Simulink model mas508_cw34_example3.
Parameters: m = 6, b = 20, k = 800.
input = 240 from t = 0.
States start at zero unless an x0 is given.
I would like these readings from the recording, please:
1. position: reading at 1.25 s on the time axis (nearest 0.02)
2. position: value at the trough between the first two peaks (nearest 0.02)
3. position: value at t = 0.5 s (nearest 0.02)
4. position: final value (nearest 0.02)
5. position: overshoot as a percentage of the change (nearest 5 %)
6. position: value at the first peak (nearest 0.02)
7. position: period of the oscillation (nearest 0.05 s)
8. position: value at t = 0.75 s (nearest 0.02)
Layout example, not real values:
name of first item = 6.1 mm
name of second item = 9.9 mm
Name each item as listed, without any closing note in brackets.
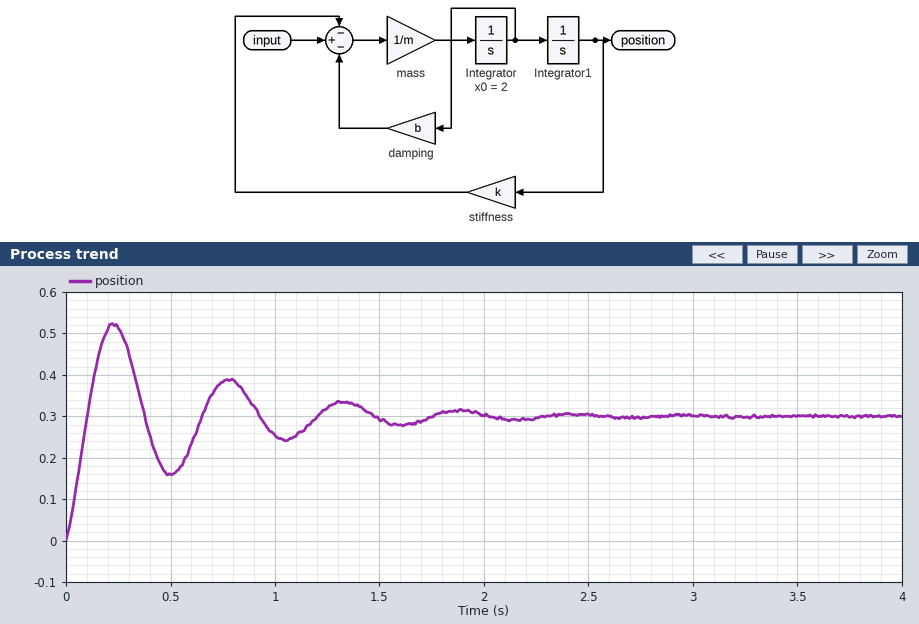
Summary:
position: reading at 1.25 s on the time axis = 0.32
position: value at the trough between the first two peaks = 0.16
position: value at t = 0.5 s = 0.16
position: final value = 0.30
position: overshoot as a percentage of the change = 75 %
position: value at the first peak = 0.52
position: period of the oscillation = 0.55 s
position: value at t = 0.75 s = 0.38
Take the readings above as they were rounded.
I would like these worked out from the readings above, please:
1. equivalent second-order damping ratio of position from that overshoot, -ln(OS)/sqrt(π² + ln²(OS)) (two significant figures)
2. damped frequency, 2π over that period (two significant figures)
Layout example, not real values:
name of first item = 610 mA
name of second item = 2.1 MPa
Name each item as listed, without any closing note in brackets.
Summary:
equivalent second-order damping ratio of position from that overshoot, -ln(OS)/sqrt(π² + ln²(OS)) = 0.091
damped frequency, 2π over that period = 11 rad/s
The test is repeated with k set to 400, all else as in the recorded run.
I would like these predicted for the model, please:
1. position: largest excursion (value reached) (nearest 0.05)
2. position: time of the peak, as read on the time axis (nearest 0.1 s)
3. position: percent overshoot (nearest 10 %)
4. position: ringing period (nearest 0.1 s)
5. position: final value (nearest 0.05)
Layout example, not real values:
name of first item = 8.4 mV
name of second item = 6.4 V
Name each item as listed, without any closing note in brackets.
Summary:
position: largest excursion (value reached) = 0.95
position: time of the peak, as read on the time axis = 0.3 s
position: percent overshoot = 60 %
position: ringing period = 0.8 s
position: final value = 0.60
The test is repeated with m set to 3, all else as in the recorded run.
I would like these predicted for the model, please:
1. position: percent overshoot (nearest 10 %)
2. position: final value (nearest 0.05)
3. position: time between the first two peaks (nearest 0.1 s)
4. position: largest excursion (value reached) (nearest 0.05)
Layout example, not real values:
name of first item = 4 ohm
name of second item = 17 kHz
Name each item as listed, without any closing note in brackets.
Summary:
position: percent overshoot = 60 %
position: final value = 0.30
position: time between the first two peaks = 0.4 s
position: largest excursion (value reached) = 0.45
